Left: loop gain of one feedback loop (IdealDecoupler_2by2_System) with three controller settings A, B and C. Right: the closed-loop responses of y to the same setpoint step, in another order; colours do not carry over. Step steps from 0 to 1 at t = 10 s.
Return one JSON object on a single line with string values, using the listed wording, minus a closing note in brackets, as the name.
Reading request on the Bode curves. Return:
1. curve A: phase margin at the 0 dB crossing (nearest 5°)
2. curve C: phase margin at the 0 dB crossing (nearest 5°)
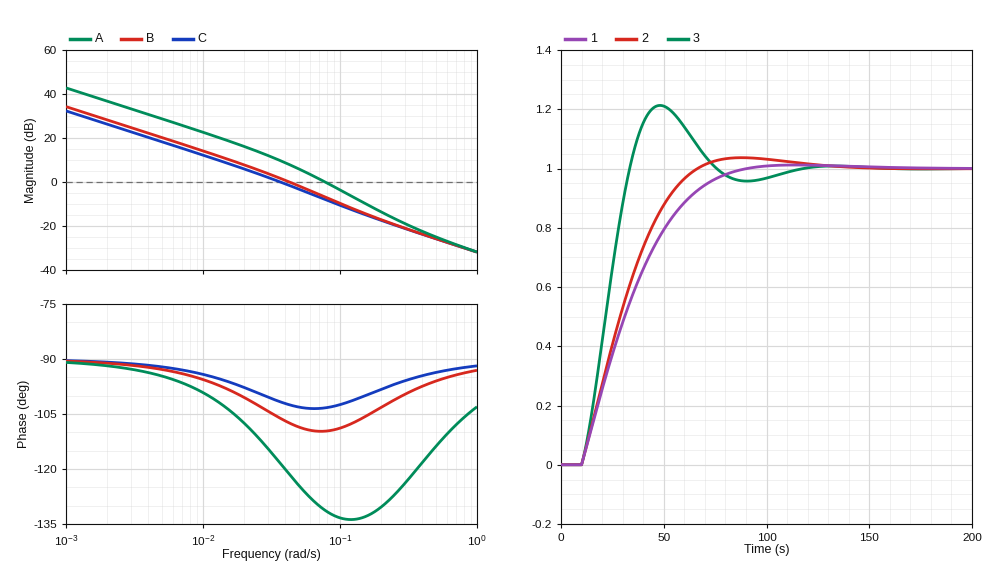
{"curve A: phase margin at the 0 dB crossing": "50°", "curve C: phase margin at the 0 dB crossing": "80°"}
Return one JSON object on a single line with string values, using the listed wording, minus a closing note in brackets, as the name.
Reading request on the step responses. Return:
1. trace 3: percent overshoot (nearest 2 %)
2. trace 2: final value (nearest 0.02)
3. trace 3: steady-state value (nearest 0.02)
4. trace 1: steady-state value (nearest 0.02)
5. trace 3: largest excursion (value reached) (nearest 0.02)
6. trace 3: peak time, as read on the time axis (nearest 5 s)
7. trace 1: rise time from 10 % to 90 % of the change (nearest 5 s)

{"trace 3: percent overshoot": "22 %", "trace 2: final value": "1.00", "trace 3: steady-state value": "1.00", "trace 1: steady-state value": "1.00", "trace 3: largest excursion (value reached)": "1.22", "trace 3: peak time, as read on the time axis": "50 s", "trace 1: rise time from 10 % to 90 % of the change": "50 s"}
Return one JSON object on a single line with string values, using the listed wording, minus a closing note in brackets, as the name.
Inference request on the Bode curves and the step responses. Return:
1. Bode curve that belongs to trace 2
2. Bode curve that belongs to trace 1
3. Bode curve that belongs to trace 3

{"Bode curve that belongs to trace 2": "B", "Bode curve that belongs to trace 1": "C", "Bode curve that belongs to trace 3": "A"}
